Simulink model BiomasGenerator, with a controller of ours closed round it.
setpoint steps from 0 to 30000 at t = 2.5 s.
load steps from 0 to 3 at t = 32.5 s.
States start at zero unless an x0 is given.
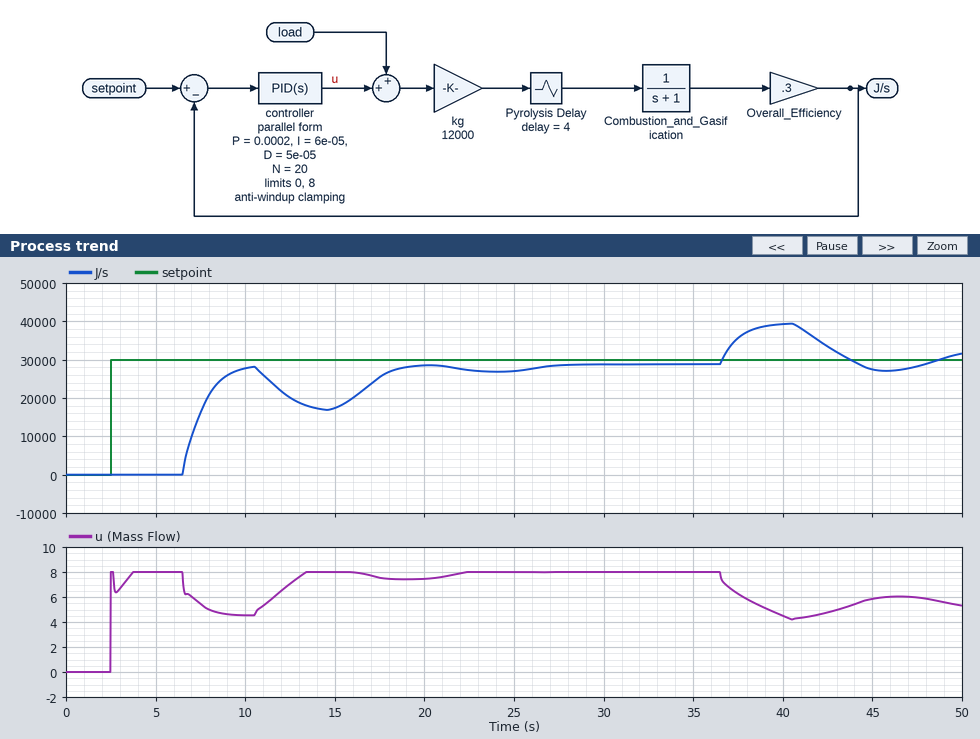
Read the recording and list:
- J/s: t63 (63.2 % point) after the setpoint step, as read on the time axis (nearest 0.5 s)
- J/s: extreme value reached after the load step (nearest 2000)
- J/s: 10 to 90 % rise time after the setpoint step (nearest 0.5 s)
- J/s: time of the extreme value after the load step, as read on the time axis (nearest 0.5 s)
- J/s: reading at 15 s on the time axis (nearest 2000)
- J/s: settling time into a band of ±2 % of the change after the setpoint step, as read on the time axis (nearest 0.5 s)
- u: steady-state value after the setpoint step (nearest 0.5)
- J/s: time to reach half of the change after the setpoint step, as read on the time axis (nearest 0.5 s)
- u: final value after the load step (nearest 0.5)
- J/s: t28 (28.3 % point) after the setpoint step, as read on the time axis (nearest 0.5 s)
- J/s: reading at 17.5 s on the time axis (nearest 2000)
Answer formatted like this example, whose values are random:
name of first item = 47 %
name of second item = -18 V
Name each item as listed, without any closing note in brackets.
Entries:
J/s: t63 (63.2 % point) after the setpoint step, as read on the time axis = 7.5 s
J/s: extreme value reached after the load step = 40000
J/s: 10 to 90 % rise time after the setpoint step = 2.5 s
J/s: time of the extreme value after the load step, as read on the time axis = 40.5 s
J/s: reading at 15 s on the time axis = 18000
J/s: settling time into a band of ±2 % of the change after the setpoint step, as read on the time axis = 27.0 s
u: steady-state value after the setpoint step = 8.0
J/s: time to reach half of the change after the setpoint step, as read on the time axis = 7.5 s
u: final value after the load step = 5.5
J/s: t28 (28.3 % point) after the setpoint step, as read on the time axis = 7.0 s
J/s: reading at 17.5 s on the time axis = 26000
